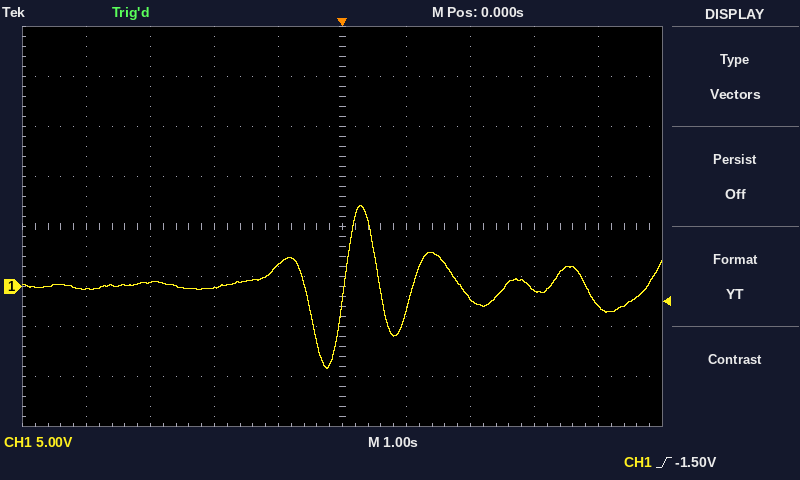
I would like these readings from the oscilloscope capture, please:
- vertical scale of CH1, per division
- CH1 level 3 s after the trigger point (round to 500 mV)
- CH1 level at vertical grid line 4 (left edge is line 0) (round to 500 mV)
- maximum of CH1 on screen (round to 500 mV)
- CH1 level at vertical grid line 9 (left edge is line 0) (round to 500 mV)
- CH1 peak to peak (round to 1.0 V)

5 V
-500 mV
2.0 V
8.0 V
-2.0 V
16.0 V
